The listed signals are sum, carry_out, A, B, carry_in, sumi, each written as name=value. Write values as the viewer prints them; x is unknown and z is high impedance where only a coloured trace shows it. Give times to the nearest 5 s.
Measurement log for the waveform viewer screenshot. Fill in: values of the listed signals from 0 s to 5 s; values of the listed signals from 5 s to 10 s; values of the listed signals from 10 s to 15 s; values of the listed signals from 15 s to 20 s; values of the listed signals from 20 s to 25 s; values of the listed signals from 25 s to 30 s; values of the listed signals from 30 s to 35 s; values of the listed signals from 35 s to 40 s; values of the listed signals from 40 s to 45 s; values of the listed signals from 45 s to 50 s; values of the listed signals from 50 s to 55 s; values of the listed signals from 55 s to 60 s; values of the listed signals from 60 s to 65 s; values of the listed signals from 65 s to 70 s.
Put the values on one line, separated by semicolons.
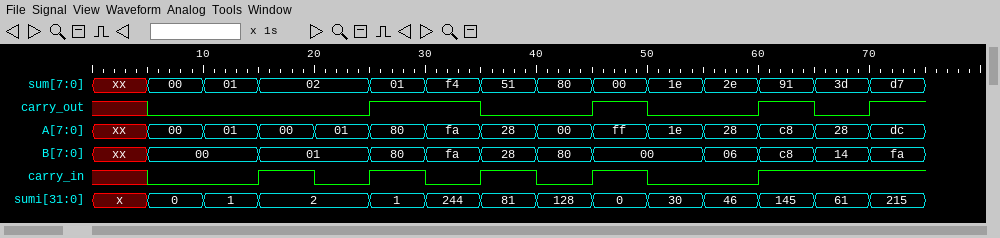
sum=xx, carry_out=x, A=xx, B=xx, carry_in=x, sumi=x; sum=00, carry_out=0, A=00, B=00, carry_in=0, sumi=0; sum=01, carry_out=0, A=01, B=00, carry_in=0, sumi=1; sum=02, carry_out=0, A=00, B=01, carry_in=1, sumi=2; sum=02, carry_out=0, A=01, B=01, carry_in=0, sumi=2; sum=01, carry_out=1, A=80, B=80, carry_in=1, sumi=1; sum=f4, carry_out=1, A=fa, B=fa, carry_in=0, sumi=244; sum=51, carry_out=0, A=28, B=28, carry_in=1, sumi=81; sum=80, carry_out=0, A=00, B=80, carry_in=0, sumi=128; sum=00, carry_out=1, A=ff, B=00, carry_in=1, sumi=0; sum=1e, carry_out=0, A=1e, B=00, carry_in=0, sumi=30; sum=2e, carry_out=0, A=28, B=06, carry_in=0, sumi=46; sum=91, carry_out=1, A=c8, B=c8, carry_in=1, sumi=145; sum=3d, carry_out=0, A=28, B=14, carry_in=1, sumi=61
